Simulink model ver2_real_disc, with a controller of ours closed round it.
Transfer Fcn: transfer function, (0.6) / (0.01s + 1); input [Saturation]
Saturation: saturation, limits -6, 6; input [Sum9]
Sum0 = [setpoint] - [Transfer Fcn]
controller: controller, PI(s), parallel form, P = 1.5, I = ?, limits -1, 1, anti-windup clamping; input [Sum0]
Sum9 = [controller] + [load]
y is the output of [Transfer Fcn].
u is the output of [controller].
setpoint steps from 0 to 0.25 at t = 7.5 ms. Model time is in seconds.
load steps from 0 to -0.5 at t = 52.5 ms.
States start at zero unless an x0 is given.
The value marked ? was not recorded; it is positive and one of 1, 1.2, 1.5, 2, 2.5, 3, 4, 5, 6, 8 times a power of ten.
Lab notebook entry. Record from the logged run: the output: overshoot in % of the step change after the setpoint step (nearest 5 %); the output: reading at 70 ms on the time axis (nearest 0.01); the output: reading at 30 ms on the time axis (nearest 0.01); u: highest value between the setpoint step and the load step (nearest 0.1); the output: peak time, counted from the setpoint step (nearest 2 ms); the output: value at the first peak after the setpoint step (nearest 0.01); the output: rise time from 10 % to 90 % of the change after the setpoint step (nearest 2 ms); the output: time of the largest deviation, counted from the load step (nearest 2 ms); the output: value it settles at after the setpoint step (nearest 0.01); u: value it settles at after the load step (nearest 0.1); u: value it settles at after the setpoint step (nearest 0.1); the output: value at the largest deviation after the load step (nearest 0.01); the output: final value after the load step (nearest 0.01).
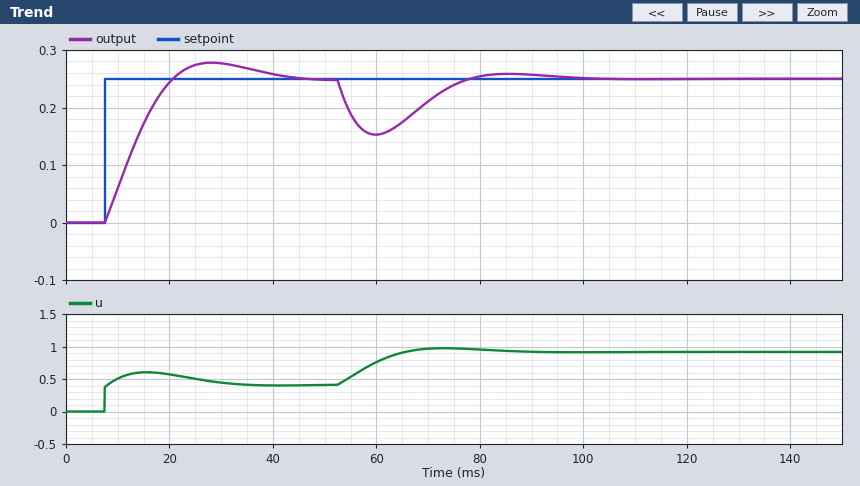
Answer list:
10 %
0.21
0.28
0.6
20 ms
0.28
10 ms
8 ms
0.25
0.9
0.4
0.15
0.25
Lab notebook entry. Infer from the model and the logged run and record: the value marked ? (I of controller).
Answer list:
400
